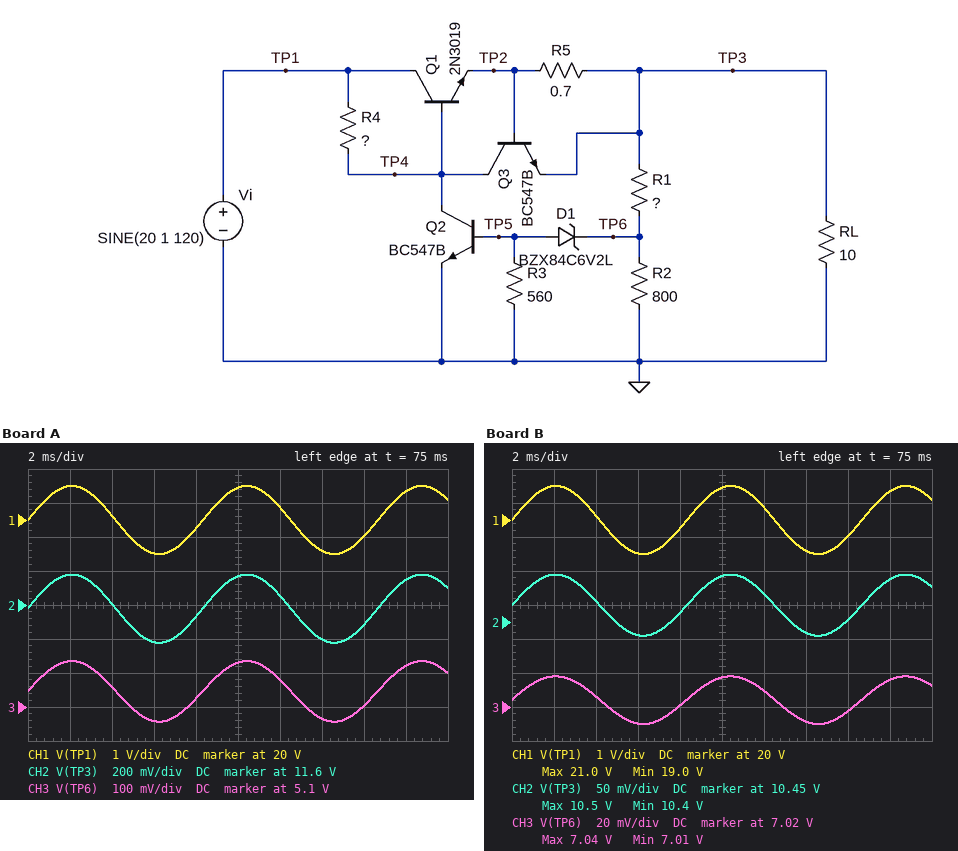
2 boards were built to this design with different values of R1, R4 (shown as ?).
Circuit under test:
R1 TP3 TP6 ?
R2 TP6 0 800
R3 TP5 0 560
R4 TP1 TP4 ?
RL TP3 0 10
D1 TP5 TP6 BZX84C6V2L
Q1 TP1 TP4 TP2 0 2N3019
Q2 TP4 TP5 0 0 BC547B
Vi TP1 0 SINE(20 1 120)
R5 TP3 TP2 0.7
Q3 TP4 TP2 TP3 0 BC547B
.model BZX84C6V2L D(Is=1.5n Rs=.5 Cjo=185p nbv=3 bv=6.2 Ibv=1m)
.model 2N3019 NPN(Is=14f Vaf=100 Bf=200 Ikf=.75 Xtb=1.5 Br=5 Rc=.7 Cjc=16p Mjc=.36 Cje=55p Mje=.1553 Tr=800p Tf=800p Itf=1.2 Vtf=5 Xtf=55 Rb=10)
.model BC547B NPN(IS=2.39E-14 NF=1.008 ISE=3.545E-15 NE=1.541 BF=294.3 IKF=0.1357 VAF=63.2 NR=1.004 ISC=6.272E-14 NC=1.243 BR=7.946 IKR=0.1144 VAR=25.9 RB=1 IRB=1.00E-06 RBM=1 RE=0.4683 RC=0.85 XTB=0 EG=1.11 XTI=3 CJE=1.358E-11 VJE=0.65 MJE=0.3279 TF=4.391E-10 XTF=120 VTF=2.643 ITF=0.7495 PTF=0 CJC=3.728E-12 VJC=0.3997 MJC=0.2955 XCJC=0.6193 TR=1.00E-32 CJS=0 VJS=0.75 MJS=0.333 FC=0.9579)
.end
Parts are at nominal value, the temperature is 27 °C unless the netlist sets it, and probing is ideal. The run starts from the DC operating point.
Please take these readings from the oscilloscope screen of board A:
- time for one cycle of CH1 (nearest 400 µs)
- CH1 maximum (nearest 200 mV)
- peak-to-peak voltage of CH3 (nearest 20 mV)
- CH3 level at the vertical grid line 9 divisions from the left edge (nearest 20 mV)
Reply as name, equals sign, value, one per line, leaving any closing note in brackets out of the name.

time for one cycle of CH1 = 8.4 ms
CH1 maximum = 21.0 V
peak-to-peak voltage of CH3 = 180 mV
CH3 level at the vertical grid line 9 divisions from the left edge = 5.22 V
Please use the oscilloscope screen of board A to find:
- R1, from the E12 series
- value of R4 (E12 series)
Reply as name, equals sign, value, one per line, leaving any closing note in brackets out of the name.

R1, from the E12 series = 1 kΩ
value of R4 = 100 Ω
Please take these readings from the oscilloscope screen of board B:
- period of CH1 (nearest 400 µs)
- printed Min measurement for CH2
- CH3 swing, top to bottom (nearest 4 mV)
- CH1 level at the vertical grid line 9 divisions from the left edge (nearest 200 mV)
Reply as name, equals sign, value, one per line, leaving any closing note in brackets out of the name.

period of CH1 = 8.4 ms
printed Min measurement for CH2 = 10.4 V
CH3 swing, top to bottom = 28 mV
CH1 level at the vertical grid line 9 divisions from the left edge = 20.8 V
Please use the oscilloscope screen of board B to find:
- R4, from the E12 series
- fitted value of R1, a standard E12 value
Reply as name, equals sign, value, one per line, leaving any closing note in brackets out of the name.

R4, from the E12 series = 82 Ω
fitted value of R1, a standard E12 value = 330 Ω
